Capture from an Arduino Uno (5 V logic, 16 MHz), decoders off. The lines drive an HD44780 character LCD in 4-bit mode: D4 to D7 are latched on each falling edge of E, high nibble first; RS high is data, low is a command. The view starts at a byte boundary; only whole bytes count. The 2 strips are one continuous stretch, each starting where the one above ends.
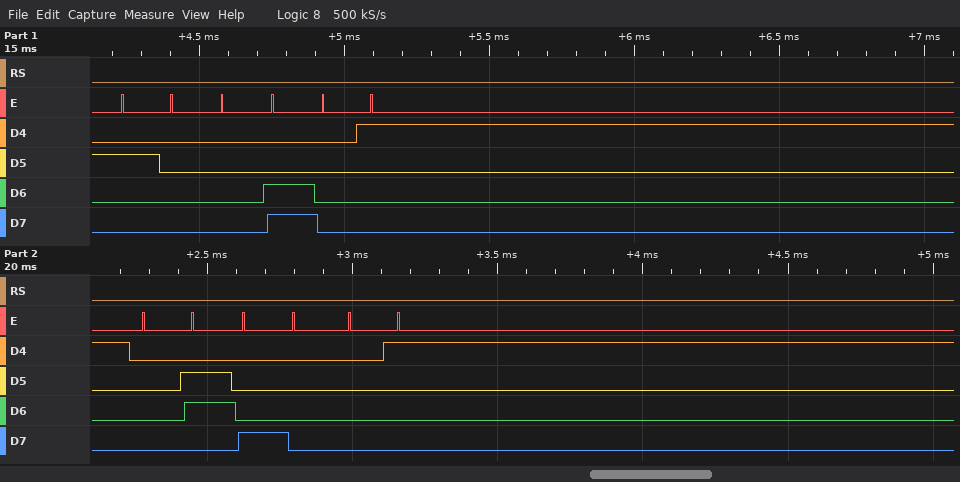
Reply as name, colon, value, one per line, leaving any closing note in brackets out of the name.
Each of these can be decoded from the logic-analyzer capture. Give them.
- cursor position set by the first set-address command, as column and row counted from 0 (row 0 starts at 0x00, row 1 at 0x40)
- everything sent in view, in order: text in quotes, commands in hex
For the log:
cursor position set by the first set-address command, as column and row counted from 0: column 0, row 0
everything sent in view, in order: text in quotes, commands in hex: 0x20 0x0C 0x01 0x06 0x80 0x01
